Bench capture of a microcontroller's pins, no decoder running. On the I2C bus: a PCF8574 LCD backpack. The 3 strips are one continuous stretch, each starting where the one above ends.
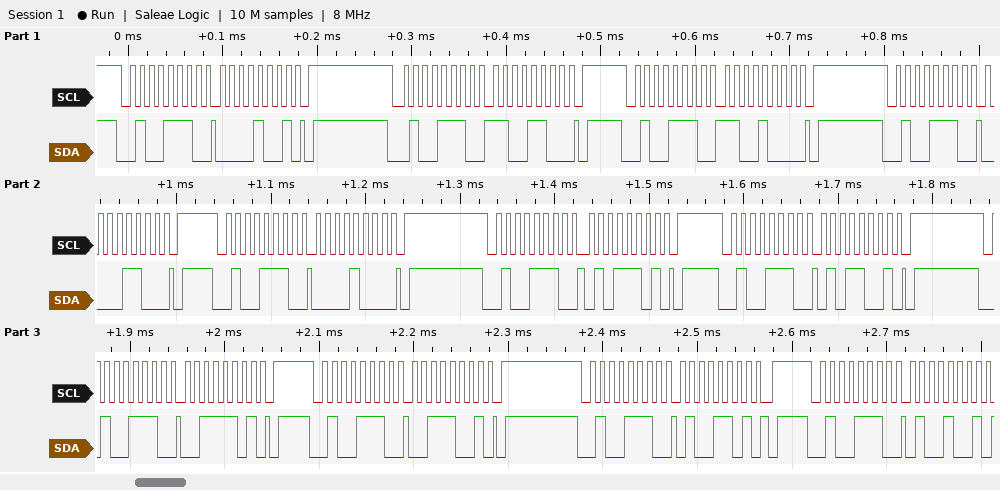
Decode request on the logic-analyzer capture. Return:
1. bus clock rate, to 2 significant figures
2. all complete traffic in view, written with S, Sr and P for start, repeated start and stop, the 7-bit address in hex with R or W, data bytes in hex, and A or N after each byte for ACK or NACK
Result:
100 kHz
S 27W A 09 A P S 27W A CC A P S 27W A C8 A P S 27W A 0C A P S 27W A 08 A P S 27W A 5D A P S 27W A 59 A P S 27W A 3D A P S 27W A 39 A P S 27W A 4D A P S 27W A 49 A
